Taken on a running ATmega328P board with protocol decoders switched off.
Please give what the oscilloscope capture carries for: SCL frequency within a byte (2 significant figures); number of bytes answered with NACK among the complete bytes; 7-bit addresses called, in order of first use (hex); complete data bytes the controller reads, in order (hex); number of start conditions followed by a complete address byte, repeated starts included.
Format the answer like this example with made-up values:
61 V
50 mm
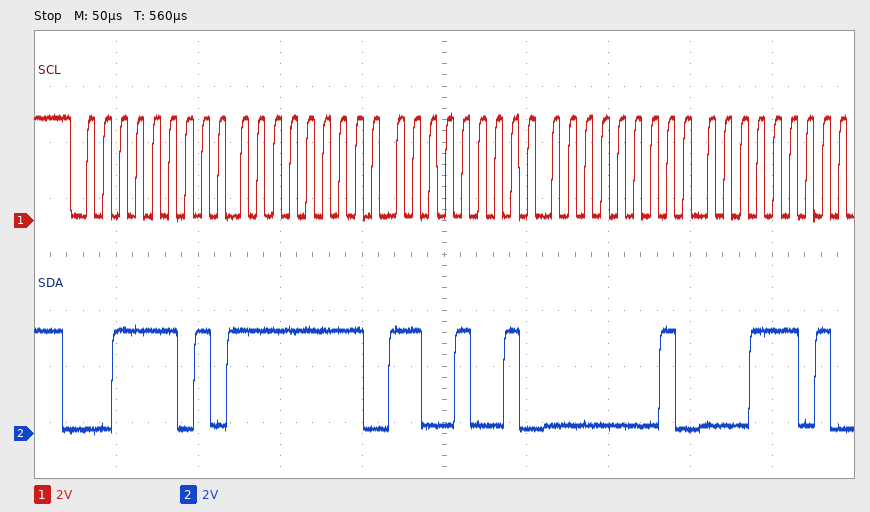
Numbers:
100 kHz
0
0x1E
FF C9 01 1D
1
